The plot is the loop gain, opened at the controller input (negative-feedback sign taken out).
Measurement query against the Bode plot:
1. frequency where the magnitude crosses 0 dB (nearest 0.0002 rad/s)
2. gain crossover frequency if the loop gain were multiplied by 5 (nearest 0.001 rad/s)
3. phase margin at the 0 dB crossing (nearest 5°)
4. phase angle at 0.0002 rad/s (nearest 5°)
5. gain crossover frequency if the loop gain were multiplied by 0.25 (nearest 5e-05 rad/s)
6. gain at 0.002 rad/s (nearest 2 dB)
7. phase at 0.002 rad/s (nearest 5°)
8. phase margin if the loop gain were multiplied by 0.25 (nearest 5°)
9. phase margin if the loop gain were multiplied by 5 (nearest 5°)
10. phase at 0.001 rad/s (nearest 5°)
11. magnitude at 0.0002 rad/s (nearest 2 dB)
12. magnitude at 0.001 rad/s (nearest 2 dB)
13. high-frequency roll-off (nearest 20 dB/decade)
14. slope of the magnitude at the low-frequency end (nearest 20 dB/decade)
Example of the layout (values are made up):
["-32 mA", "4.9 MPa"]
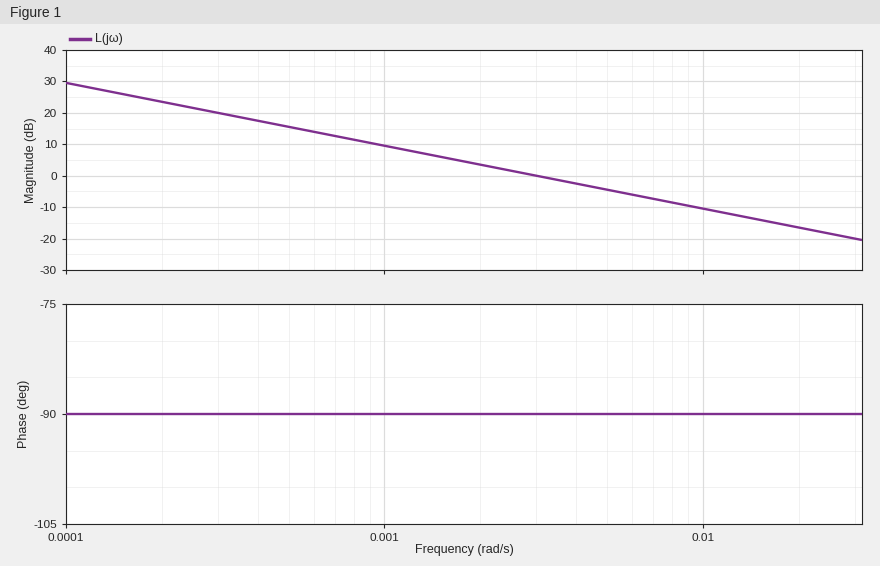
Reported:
["0.0030 rad/s", "0.015 rad/s", "90°", "-90°", "0.00075 rad/s", "4 dB", "-90°", "90°", "90°", "-90°", "24 dB", "10 dB", "-20 dB/decade", "-20 dB/decade"]
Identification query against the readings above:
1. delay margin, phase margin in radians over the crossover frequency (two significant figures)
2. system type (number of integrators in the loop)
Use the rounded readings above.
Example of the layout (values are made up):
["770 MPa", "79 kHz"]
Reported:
["520 s", "1"]
